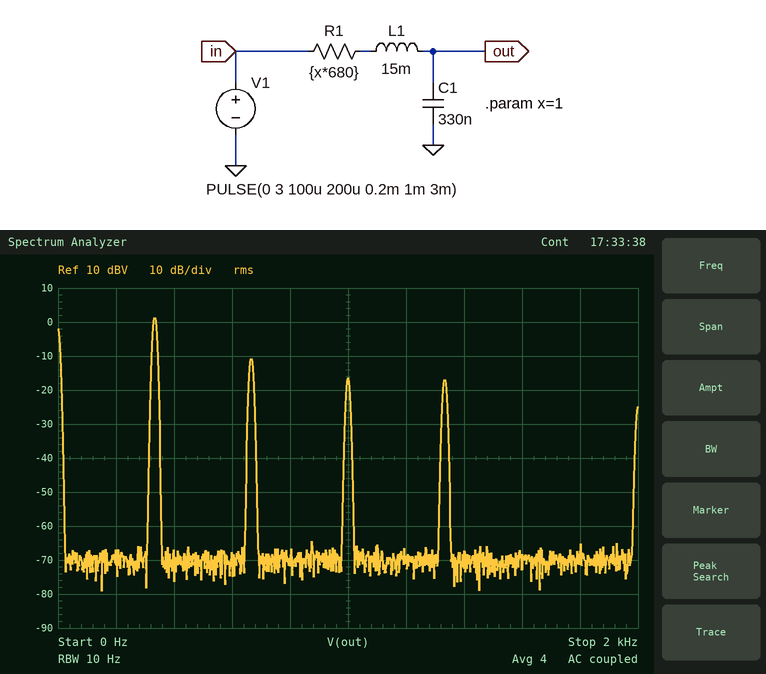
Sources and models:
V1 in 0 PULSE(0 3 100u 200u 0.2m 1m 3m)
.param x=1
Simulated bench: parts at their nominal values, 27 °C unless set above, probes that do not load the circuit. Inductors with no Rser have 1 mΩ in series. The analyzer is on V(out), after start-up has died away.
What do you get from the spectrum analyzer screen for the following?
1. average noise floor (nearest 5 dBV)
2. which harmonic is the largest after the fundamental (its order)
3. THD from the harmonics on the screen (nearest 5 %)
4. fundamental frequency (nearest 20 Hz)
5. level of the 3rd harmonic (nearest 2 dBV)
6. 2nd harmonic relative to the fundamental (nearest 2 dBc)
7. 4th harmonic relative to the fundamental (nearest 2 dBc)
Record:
-70 dBV
2
30 %
340 Hz
-16 dBV
-12 dBc
-18 dBc
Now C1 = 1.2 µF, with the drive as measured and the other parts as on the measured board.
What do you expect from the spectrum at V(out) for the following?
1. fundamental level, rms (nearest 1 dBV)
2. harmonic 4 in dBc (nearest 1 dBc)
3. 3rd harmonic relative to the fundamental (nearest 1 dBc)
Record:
-4 dBV
-24 dBc
-23 dBc
